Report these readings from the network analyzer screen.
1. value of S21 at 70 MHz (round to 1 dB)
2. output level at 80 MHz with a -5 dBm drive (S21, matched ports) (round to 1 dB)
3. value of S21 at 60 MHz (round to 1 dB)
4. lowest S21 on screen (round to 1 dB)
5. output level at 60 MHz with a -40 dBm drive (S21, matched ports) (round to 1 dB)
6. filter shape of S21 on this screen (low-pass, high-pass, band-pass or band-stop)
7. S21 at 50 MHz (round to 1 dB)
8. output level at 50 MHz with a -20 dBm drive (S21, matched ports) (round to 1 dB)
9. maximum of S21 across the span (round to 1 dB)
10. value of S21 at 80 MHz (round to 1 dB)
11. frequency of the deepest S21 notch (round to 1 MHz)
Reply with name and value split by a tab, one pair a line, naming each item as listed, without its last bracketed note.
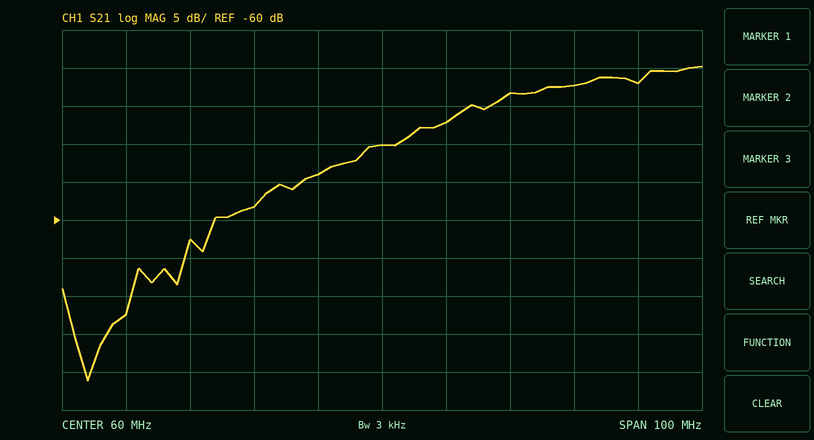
value of S21 at 70 MHz	-47 dB
output level at 80 MHz with a -5 dBm drive (S21, matched ports)	-48 dBm
value of S21 at 60 MHz	-50 dB
lowest S21 on screen	-81 dB
output level at 60 MHz with a -40 dBm drive (S21, matched ports)	-90 dBm
filter shape of S21 on this screen	high-pass
S21 at 50 MHz	-54 dB
output level at 50 MHz with a -20 dBm drive (S21, matched ports)	-74 dBm
maximum of S21 across the span	-40 dB
value of S21 at 80 MHz	-43 dB
frequency of the deepest S21 notch	14 MHz
